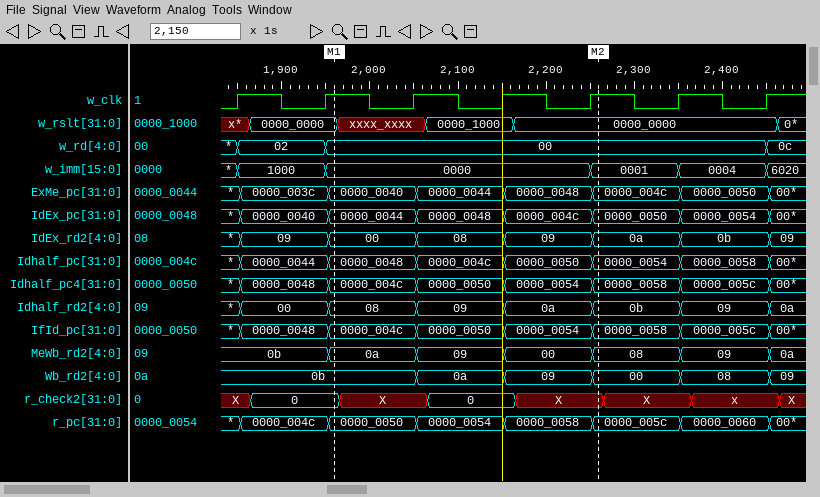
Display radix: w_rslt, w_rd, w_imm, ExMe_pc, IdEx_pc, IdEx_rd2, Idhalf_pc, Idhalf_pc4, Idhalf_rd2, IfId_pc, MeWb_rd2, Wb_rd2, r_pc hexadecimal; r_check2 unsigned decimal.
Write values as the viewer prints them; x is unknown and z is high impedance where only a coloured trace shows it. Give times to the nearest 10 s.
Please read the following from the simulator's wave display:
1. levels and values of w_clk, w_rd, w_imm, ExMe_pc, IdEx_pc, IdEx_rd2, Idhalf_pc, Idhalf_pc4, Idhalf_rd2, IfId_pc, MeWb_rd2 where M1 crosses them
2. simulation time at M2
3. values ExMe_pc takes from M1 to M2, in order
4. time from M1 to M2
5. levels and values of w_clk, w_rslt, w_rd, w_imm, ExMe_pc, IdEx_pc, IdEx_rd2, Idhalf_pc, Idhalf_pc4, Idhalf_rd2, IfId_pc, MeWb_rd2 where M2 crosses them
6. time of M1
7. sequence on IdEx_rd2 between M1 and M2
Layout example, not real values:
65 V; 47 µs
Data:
w_clk=1, w_rd=00, w_imm=0000, ExMe_pc=0000_0040, IdEx_pc=0000_0044, IdEx_rd2=00, Idhalf_pc=0000_0048, Idhalf_pc4=0000_004c, Idhalf_rd2=08, IfId_pc=0000_004c, MeWb_rd2=0a; 2260 s; 0000_0040, 0000_0044, 0000_0048, 0000_004c; 300 s; w_clk=1, w_rslt=0000_0000, w_rd=00, w_imm=0001, ExMe_pc=0000_004c, IdEx_pc=0000_0050, IdEx_rd2=0a, Idhalf_pc=0000_0054, Idhalf_pc4=0000_0058, Idhalf_rd2=0b, IfId_pc=0000_0058, MeWb_rd2=08; 1960 s; 00, 08, 09, 0a
